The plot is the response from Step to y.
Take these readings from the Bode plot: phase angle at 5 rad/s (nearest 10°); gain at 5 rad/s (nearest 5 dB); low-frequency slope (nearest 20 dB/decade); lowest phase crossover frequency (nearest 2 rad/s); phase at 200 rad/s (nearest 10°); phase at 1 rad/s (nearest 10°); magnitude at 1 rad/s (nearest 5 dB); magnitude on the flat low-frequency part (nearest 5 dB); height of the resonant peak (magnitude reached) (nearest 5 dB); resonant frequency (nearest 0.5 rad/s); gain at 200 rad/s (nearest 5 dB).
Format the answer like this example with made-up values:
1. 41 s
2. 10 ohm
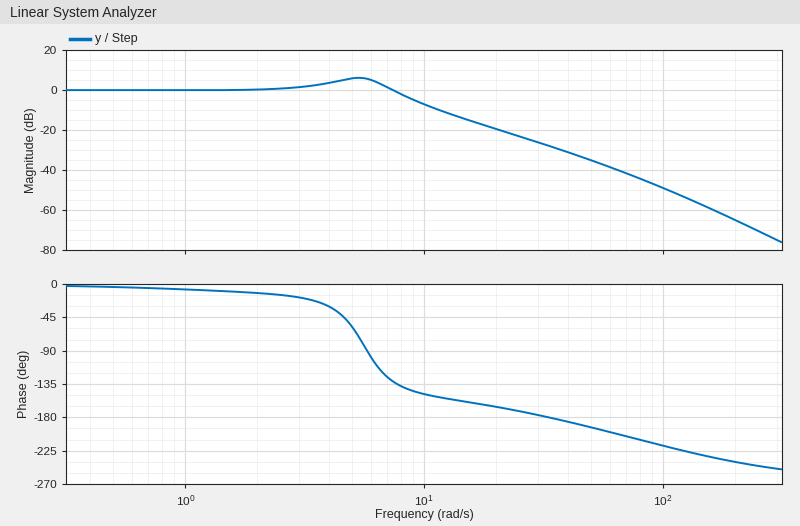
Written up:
1. -60°
2. 5 dB
3. 0 dB/decade
4. 34 rad/s
5. -240°
6. -10°
7. 0 dB
8. 0 dB
9. 5 dB
10. 5.5 rad/s
11. -65 dB
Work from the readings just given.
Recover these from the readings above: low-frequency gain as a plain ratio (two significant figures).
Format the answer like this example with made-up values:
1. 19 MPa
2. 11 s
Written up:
1. 1.0
